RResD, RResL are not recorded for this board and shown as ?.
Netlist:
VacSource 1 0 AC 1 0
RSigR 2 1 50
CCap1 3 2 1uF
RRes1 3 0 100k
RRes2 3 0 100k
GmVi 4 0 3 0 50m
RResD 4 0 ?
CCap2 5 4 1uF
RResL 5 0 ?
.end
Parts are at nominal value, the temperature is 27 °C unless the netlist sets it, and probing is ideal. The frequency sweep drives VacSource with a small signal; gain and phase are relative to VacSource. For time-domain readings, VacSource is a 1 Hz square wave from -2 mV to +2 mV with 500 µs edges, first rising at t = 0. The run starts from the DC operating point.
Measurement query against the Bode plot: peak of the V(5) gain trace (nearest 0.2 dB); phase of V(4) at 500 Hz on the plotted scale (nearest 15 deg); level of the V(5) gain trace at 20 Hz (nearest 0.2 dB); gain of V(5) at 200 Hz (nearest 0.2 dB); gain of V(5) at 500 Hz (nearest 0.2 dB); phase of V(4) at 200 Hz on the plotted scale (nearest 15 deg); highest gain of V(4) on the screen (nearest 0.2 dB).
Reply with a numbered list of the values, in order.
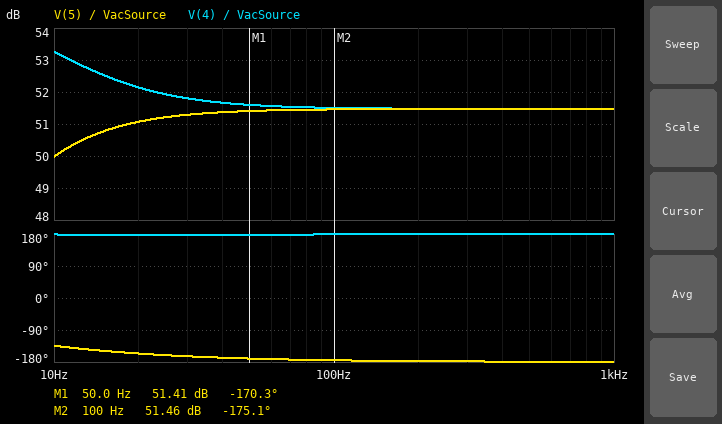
1. 51.4 dB
2. 180 deg
3. 51.0 dB
4. 51.4 dB
5. 51.4 dB
6. 180 deg
7. 53.2 dB
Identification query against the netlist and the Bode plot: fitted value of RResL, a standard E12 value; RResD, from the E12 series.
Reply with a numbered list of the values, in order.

1. 15 kΩ
2. 15 kΩ
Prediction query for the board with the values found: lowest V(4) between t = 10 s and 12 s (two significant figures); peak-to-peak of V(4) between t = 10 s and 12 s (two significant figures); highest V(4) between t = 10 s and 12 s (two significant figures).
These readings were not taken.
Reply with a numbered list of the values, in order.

1. -1.6 V
2. 3.2 V
3. 1.6 V
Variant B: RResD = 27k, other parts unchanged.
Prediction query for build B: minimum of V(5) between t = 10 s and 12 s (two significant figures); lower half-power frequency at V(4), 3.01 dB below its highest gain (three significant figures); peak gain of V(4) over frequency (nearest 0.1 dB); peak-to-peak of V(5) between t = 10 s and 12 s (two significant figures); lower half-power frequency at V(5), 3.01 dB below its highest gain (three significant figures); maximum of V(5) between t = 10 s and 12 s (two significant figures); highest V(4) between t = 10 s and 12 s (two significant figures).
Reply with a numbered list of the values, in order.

1. -1.9 V
2. 1.53 Hz
3. 57.8 dB
4. 3.8 V
5. 5.42 Hz
6. 1.9 V
7. 2.4 V
